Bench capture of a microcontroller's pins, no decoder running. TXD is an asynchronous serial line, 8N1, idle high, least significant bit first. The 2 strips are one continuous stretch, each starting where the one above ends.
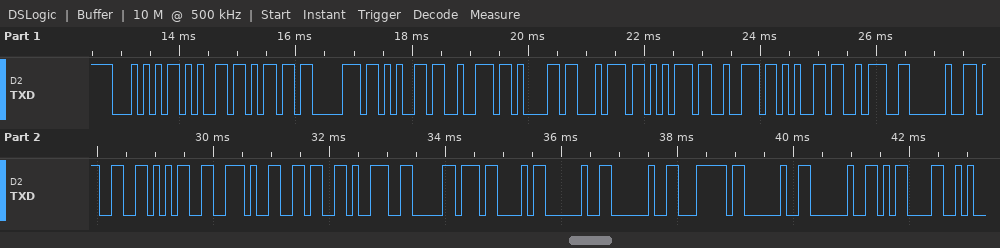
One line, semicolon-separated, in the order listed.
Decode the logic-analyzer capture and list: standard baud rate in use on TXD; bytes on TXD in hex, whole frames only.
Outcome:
9600 baud; 54 65 6D 70 65 72 61 74 75 72 65 3A 20 33 35 2E 36 39 B0 43 20 20 7C 20 20 0D
